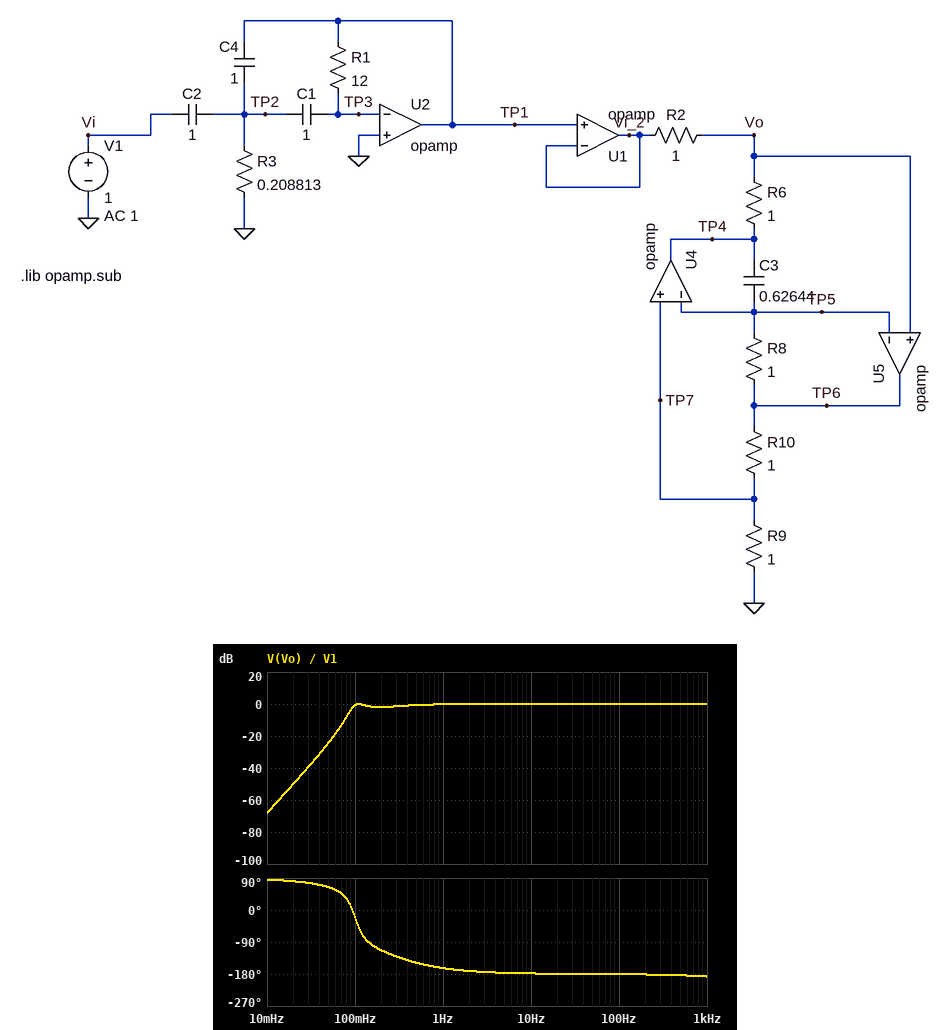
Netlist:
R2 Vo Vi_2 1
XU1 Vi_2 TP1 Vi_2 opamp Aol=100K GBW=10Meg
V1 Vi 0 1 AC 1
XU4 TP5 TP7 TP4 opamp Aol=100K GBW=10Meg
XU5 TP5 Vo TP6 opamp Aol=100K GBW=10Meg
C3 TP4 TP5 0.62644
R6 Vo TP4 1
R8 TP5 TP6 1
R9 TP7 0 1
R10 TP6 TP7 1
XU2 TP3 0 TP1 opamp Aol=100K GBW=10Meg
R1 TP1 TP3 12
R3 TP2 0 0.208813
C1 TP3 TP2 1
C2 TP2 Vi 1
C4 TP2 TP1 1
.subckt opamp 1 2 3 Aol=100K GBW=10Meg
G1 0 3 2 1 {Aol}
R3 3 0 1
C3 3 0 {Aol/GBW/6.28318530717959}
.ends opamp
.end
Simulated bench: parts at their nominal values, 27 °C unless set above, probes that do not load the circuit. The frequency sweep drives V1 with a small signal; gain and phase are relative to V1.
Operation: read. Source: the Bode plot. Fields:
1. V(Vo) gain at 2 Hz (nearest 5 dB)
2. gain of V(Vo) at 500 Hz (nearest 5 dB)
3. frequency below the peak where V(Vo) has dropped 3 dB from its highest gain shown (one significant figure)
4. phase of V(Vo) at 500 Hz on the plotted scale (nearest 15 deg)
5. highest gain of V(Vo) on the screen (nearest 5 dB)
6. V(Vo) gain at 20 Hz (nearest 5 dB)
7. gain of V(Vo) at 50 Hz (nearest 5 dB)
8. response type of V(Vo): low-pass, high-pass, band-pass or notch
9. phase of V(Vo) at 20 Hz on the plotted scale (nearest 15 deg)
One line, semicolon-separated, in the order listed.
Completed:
0 dB; 0 dB; 90 mHz; -180 deg; 0 dB; 0 dB; 0 dB; high-pass; -180 deg
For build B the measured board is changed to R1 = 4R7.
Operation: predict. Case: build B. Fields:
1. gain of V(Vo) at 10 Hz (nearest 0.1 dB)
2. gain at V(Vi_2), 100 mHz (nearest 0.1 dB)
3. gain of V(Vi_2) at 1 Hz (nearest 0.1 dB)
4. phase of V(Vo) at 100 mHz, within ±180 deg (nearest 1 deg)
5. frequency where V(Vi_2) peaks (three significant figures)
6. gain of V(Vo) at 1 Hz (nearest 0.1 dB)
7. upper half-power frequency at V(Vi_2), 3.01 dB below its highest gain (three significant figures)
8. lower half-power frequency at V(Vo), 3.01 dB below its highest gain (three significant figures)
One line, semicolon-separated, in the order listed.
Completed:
0 dB; -5.5 dB; 0.2 dB; 36 deg; 180 mHz; -0.1 dB; 359 mHz; 148 mHz
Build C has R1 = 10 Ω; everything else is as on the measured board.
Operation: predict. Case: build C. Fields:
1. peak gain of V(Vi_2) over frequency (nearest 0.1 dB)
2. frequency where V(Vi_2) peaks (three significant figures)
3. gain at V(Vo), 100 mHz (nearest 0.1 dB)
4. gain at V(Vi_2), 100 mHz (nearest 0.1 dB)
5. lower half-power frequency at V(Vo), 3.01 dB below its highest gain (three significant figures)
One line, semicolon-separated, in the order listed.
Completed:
7.5 dB; 116 mHz; -3.1 dB; 5.6 dB; 100 mHz
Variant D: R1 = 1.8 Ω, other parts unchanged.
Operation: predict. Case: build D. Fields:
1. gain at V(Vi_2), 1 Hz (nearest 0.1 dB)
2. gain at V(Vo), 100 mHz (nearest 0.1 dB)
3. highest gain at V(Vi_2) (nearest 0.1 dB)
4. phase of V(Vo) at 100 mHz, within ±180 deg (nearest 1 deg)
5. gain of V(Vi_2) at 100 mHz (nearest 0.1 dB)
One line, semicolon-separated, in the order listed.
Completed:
0.3 dB; -24.7 dB; 1.1 dB; 44 deg; -16.0 dB
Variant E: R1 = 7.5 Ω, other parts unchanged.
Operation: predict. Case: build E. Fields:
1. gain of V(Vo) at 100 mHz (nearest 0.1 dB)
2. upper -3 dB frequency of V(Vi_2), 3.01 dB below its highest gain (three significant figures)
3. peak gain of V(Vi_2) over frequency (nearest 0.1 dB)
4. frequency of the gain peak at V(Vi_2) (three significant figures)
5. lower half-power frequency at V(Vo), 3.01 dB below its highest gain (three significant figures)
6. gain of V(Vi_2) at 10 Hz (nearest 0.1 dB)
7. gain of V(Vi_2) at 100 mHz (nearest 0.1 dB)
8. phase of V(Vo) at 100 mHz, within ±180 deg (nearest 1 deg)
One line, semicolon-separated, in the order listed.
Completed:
-7.7 dB; 204 mHz; 6.3 dB; 136 mHz; 116 mHz; 0 dB; 1.0 dB; 23 deg
